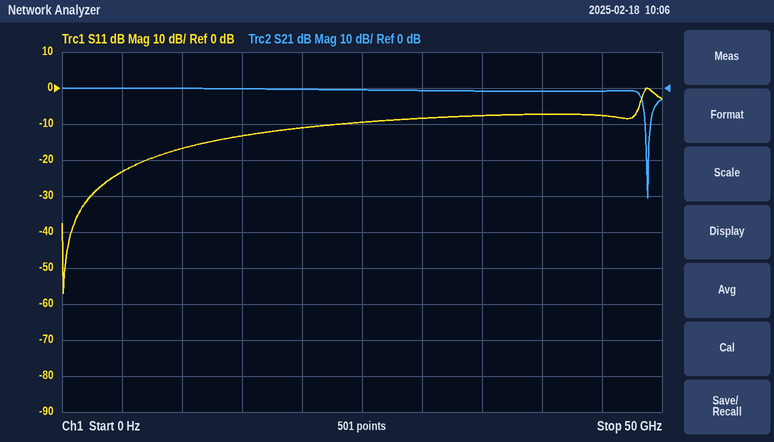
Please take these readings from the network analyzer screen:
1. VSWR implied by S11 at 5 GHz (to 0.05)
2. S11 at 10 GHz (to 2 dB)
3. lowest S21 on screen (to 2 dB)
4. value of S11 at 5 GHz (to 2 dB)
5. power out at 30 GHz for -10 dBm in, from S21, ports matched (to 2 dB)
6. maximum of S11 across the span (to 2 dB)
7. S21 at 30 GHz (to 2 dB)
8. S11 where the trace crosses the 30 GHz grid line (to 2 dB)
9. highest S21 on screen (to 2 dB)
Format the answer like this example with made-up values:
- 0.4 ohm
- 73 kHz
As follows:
- 1.15
- -16 dB
- -30 dB
- -24 dB
- -10 dBm
- 0 dB
- 0 dB
- -8 dB
- 0 dB
